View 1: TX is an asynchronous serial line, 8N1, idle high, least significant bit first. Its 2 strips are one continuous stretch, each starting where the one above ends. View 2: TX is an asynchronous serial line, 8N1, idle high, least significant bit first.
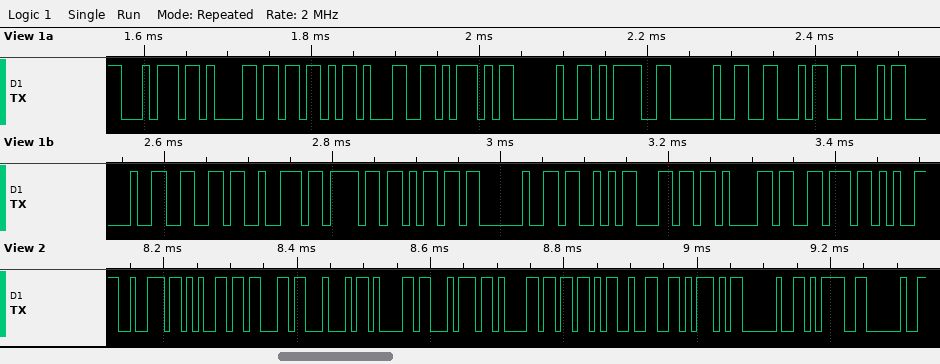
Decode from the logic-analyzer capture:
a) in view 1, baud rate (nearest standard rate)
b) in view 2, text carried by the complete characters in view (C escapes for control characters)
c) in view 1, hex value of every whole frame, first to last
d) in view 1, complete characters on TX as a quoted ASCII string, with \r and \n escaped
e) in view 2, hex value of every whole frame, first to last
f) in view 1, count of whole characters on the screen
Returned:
115200 baud
"recData[2] = "
74 61 5B 31 5D 20 3D 20 46 46 20 66 72 6F 6D 20 53 6C 61 76
"ta[1] = FF from Slav"
72 65 63 44 61 74 61 5B 32 5D 20 3D 20
20
